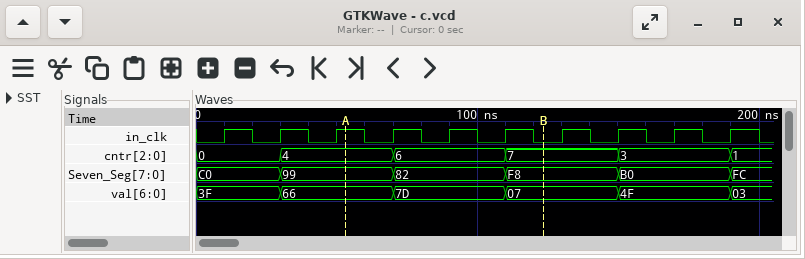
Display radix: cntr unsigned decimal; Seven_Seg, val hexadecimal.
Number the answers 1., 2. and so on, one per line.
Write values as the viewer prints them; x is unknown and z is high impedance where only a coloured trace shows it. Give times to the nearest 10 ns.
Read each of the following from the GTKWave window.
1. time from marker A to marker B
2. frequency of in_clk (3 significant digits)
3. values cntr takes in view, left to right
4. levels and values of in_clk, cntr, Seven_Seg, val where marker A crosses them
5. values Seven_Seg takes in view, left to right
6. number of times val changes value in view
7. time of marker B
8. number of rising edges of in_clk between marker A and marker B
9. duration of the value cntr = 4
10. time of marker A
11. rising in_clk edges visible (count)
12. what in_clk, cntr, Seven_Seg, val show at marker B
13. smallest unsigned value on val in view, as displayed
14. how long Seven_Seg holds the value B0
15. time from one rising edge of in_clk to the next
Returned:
1. 70 ns
2. 50.0 MHz
3. 0, 4, 6, 7, 3, 1
4. in_clk=1, cntr=4, Seven_Seg=99, val=66
5. C0, 99, 82, F8, B0, FC
6. 5
7. 120 ns
8. 3
9. 40 ns
10. 50 ns
11. 10
12. in_clk=0, cntr=7, Seven_Seg=F8, val=07
13. 03
14. 40 ns
15. 20 ns
